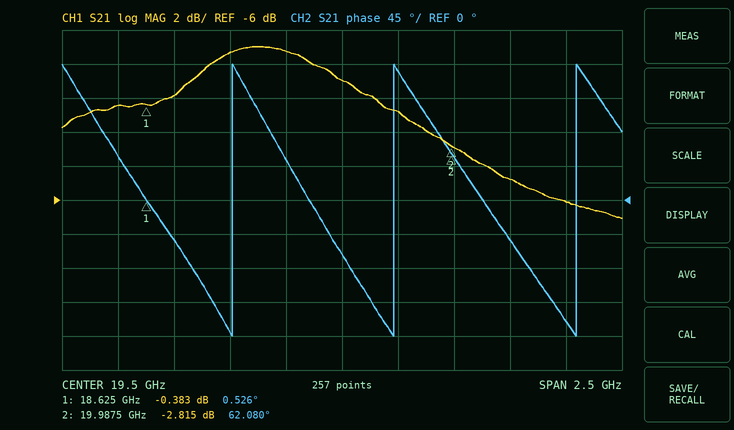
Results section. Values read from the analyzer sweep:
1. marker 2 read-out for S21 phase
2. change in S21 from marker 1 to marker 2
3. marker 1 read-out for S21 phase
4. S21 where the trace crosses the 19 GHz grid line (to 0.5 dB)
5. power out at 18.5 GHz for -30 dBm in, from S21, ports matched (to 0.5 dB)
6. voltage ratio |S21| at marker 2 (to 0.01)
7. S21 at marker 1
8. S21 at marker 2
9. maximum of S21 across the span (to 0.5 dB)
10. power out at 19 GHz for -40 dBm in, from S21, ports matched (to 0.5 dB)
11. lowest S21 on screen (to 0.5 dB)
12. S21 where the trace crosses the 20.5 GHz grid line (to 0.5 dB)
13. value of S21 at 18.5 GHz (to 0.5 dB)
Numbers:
62.080°
-2.432 dB
0.526°
2.5 dB
-30.5 dBm
0.72
-0.383 dB
-2.815 dB
3.0 dB
-37.5 dBm
-7.0 dB
-6.0 dB
-0.5 dB
